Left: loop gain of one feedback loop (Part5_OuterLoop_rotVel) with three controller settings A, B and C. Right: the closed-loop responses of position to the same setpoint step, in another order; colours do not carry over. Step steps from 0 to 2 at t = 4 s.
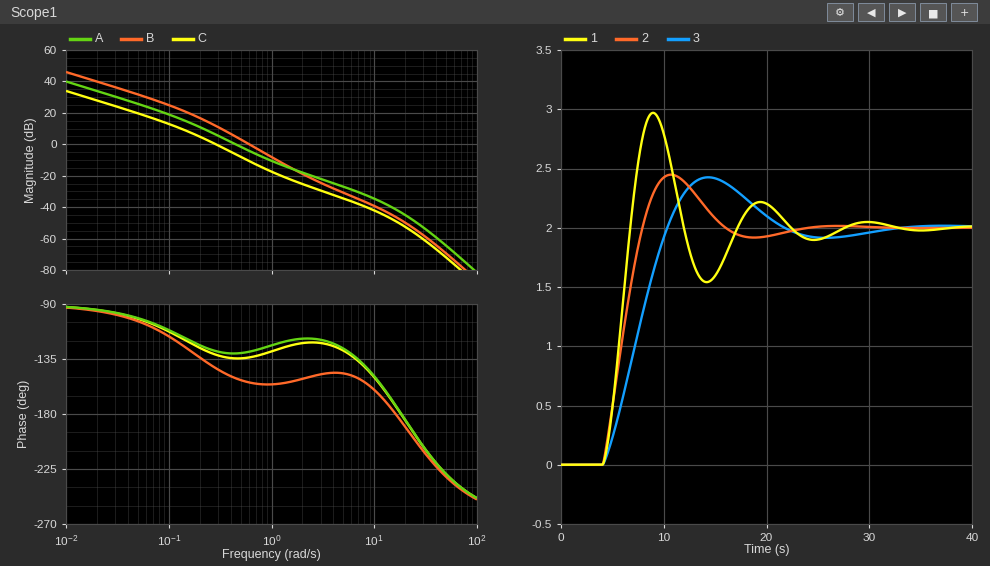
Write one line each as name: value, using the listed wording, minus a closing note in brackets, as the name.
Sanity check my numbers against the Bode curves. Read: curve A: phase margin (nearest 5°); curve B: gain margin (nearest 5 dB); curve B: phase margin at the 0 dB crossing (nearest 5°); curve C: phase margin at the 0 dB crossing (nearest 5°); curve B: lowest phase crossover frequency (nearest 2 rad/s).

curve A: phase margin: 50°
curve B: gain margin: 45 dB
curve B: phase margin at the 0 dB crossing: 25°
curve C: phase margin at the 0 dB crossing: 50°
curve B: lowest phase crossover frequency: 16 rad/s
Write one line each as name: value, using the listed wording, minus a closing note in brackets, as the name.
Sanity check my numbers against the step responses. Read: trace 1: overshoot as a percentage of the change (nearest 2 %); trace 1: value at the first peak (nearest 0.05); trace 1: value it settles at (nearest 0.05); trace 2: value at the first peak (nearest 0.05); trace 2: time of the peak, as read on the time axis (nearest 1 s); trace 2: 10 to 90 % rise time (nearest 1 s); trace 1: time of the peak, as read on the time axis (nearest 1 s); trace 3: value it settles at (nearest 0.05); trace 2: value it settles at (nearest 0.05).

trace 1: overshoot as a percentage of the change: 48 %
trace 1: value at the first peak: 2.95
trace 1: value it settles at: 2.00
trace 2: value at the first peak: 2.45
trace 2: time of the peak, as read on the time axis: 11 s
trace 2: 10 to 90 % rise time: 3 s
trace 1: time of the peak, as read on the time axis: 9 s
trace 3: value it settles at: 2.00
trace 2: value it settles at: 2.00
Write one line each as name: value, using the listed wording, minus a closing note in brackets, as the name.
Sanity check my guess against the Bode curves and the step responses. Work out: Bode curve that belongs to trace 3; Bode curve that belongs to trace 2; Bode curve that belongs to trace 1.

Bode curve that belongs to trace 3: C
Bode curve that belongs to trace 2: A
Bode curve that belongs to trace 1: B
